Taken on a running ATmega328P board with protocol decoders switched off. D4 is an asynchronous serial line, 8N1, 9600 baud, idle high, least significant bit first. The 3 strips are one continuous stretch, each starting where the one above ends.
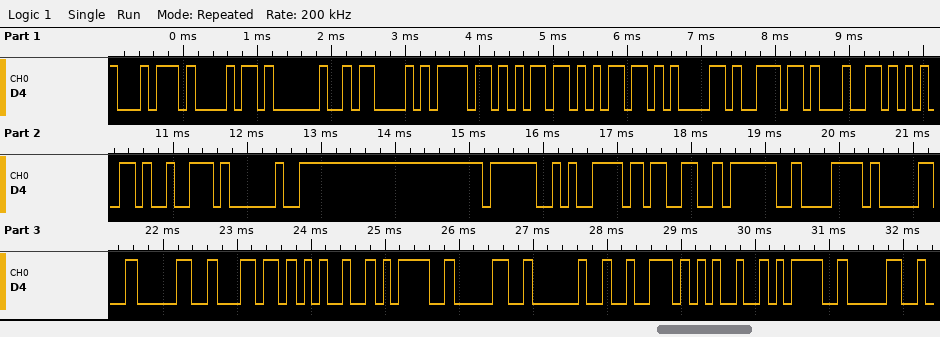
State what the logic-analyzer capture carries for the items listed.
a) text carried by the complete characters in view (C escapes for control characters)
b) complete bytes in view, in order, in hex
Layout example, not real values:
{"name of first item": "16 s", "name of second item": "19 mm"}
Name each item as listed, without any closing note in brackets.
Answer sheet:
{"text carried by the complete characters in view": "\"th Commander ?y3?x00l%=0 r%=0\"", "complete bytes in view, in order, in hex": "74 68 20 43 6F 6D 6D 61 6E 64 65 72 20 3F 79 33 3F 78 30 30 6C 25 3D 30 20 72 25 3D 30"}
